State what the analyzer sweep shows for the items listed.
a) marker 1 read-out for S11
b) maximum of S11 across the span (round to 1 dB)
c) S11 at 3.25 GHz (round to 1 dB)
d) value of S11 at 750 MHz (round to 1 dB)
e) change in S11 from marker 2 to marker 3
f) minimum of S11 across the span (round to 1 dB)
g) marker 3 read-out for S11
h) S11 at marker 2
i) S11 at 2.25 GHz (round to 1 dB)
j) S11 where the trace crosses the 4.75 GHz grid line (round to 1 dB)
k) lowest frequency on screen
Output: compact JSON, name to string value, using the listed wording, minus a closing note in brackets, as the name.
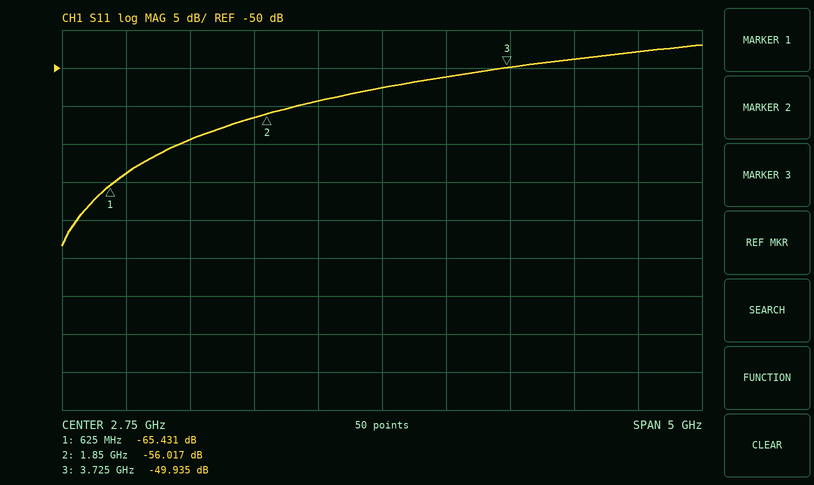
{"marker 1 read-out for S11": "-65.431 dB", "maximum of S11 across the span": "-47 dB", "S11 at 3.25 GHz": "-51 dB", "value of S11 at 750 MHz": "-64 dB", "change in S11 from marker 2 to marker 3": "6.082 dB", "minimum of S11 across the span": "-73 dB", "marker 3 read-out for S11": "-49.935 dB", "S11 at marker 2": "-56.017 dB", "S11 at 2.25 GHz": "-54 dB", "S11 where the trace crosses the 4.75 GHz grid line": "-48 dB", "lowest frequency on screen": "250 MHz"}
